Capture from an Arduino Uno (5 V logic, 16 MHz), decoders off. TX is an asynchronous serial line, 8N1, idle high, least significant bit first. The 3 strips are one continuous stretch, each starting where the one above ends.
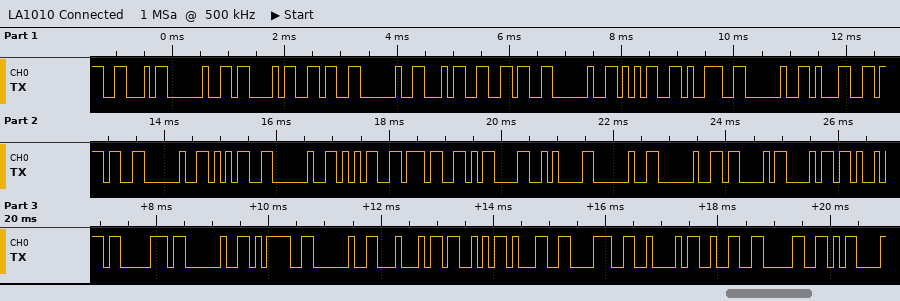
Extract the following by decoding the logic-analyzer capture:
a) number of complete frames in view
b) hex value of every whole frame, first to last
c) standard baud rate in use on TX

37
46 20 43 36 20 34 36 20 35 39 20 31 37 20 35 20 35 37 0D 0A 20 20 43 68 69 70 20 3D 20 44 53 31 38 42 32 30 0D
9600 baud
